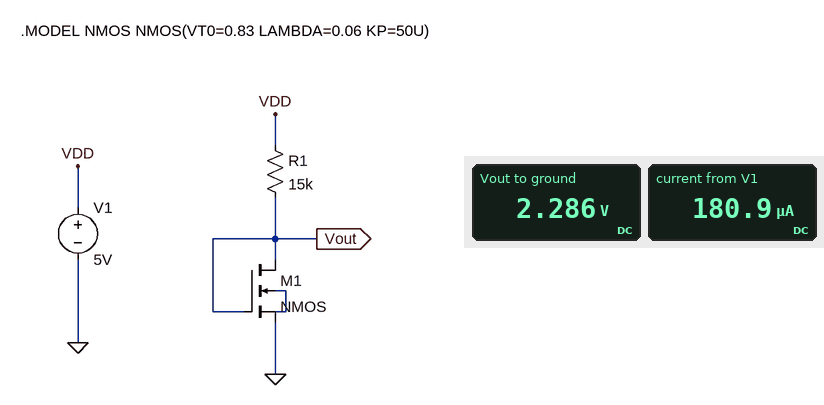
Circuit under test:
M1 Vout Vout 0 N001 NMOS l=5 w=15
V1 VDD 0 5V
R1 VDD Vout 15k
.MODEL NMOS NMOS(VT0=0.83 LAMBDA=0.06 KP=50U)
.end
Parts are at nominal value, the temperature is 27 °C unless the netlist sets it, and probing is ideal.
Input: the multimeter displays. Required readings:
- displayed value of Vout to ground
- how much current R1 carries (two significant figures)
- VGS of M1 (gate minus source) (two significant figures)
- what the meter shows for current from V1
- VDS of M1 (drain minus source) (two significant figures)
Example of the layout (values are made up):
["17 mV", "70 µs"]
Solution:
["2.286 V", "180 µA", "2.3 V", "180.9 µA", "2.3 V"]
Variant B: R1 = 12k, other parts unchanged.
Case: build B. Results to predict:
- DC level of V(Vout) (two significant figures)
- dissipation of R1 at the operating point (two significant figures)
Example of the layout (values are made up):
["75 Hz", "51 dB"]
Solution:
["2.4 V", "560 µW"]
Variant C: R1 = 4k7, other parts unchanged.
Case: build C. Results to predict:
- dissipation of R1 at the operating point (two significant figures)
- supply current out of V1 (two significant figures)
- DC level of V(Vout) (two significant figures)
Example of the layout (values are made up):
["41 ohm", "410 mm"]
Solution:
["840 µW", "420 µA", "3.0 V"]
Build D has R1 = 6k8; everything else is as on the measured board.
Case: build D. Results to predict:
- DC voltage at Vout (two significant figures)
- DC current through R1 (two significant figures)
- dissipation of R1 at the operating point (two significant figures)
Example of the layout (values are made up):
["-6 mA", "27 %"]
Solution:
["2.8 V", "330 µA", "730 µW"]
